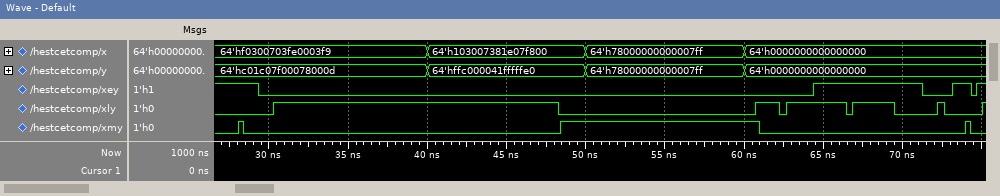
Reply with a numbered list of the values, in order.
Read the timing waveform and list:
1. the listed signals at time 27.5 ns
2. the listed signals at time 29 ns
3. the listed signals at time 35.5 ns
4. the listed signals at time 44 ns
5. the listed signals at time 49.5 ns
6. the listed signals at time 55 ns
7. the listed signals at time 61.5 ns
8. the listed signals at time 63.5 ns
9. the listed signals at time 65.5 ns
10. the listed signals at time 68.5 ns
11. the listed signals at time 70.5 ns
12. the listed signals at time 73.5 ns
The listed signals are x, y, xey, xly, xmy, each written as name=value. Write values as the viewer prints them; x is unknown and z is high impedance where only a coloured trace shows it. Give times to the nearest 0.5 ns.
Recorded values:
1. x=64'hf0300703fe0003f9, y=64'hc01c07f00078000d, xey=1, xly=0, xmy=0
2. x=64'hf0300703fe0003f9, y=64'hc01c07f00078000d, xey=1, xly=0, xmy=0
3. x=64'hf0300703fe0003f9, y=64'hc01c07f00078000d, xey=0, xly=1, xmy=0
4. x=64'h103007381e07f800, y=64'hffc000041fffffe0, xey=0, xly=1, xmy=0
5. x=64'h103007381e07f800, y=64'hffc000041fffffe0, xey=0, xly=0, xmy=1
6. x=64'h78000000000007ff, y=64'h78000000000007ff, xey=0, xly=0, xmy=1
7. x=64'h0000000000000000, y=64'h0000000000000000, xey=0, xly=1, xmy=0
8. x=64'h0000000000000000, y=64'h0000000000000000, xey=0, xly=1, xmy=0
9. x=64'h0000000000000000, y=64'h0000000000000000, xey=1, xly=1, xmy=0
10. x=64'h0000000000000000, y=64'h0000000000000000, xey=1, xly=1, xmy=0
11. x=64'h0000000000000000, y=64'h0000000000000000, xey=1, xly=0, xmy=0
12. x=64'h0000000000000000, y=64'h0000000000000000, xey=1, xly=0, xmy=0
